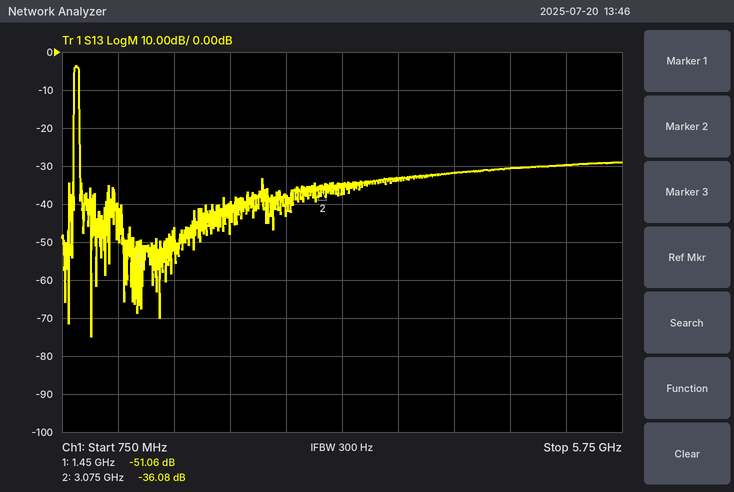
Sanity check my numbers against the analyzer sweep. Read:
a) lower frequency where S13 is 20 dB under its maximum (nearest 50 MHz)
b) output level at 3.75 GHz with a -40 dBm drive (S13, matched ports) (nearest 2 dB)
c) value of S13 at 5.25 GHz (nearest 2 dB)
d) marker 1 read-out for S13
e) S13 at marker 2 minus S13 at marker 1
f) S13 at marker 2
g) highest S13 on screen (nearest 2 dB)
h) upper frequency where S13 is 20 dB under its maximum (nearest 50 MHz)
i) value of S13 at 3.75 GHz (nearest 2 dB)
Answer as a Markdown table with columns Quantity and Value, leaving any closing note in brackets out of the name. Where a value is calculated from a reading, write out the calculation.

| Quantity | Value |
|---|---|
| lower frequency where S13 is 20 dB under its maximum | 850 MHz |
| output level at 3.75 GHz with a -40 dBm drive (S13, matched ports) | -40 dBm + (-34 dB) = -74 dBm |
| value of S13 at 5.25 GHz | -30 dB |
| marker 1 read-out for S13 | -51.06 dB |
| S13 at marker 2 minus S13 at marker 1 | -36.08 − (-51.06) = 14.98 dB |
| S13 at marker 2 | -36.08 dB |
| highest S13 on screen | -4 dB |
| upper frequency where S13 is 20 dB under its maximum | 900 MHz |
| value of S13 at 3.75 GHz | -34 dB |
